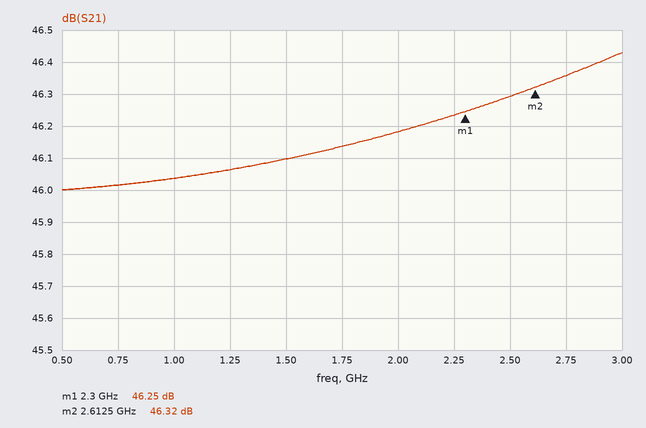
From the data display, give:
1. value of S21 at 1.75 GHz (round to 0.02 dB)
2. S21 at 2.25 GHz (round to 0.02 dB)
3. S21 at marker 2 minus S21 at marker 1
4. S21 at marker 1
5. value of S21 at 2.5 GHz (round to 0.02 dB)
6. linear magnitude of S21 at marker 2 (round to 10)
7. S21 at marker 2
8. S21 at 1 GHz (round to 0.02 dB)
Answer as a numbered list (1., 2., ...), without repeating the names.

1. 46.14 dB
2. 46.24 dB
3. 0.07 dB
4. 46.25 dB
5. 46.30 dB
6. 210
7. 46.32 dB
8. 46.04 dB
